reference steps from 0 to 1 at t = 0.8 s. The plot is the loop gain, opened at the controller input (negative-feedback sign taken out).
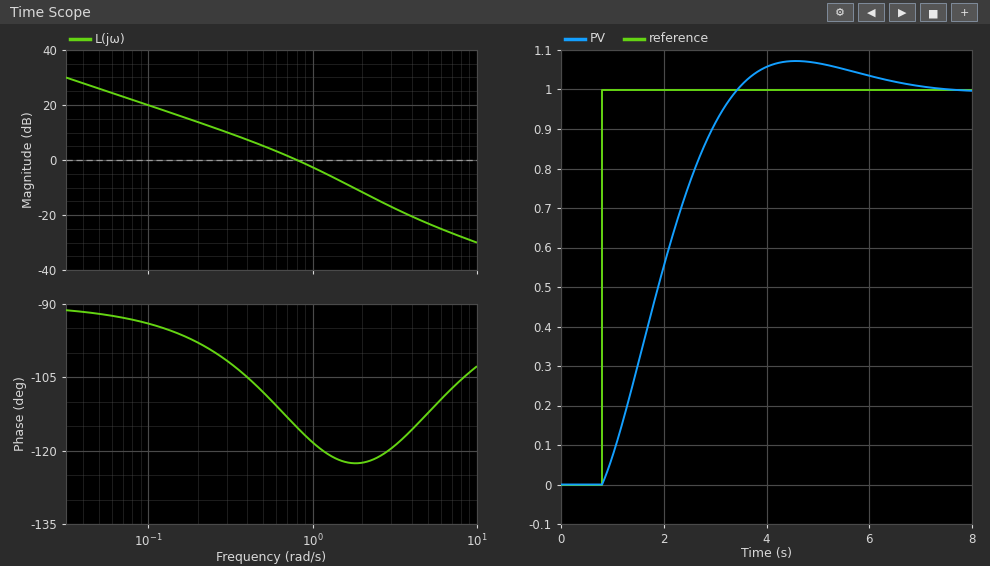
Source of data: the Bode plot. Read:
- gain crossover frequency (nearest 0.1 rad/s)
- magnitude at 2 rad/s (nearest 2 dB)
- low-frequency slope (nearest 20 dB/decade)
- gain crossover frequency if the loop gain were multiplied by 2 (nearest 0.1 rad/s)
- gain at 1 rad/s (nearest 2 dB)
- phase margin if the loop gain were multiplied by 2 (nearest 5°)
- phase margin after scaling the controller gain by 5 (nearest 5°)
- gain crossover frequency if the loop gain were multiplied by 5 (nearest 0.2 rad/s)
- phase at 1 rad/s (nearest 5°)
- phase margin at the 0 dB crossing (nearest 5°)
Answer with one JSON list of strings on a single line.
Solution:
["0.8 rad/s", "-12 dB", "-20 dB/decade", "1.3 rad/s", "-2 dB", "60°", "60°", "2.4 rad/s", "-120°", "65°"]
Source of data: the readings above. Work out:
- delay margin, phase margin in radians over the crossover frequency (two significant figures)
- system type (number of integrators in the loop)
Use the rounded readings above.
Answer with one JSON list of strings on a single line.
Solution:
["1.4 s", "1"]
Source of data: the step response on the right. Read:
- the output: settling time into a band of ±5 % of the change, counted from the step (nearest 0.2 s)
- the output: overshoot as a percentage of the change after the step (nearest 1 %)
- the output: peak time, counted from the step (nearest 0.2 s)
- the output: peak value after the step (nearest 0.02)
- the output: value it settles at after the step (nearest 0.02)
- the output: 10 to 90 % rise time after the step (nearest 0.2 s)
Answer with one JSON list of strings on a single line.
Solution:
["4.8 s", "7 %", "3.8 s", "1.08", "1.00", "1.8 s"]
